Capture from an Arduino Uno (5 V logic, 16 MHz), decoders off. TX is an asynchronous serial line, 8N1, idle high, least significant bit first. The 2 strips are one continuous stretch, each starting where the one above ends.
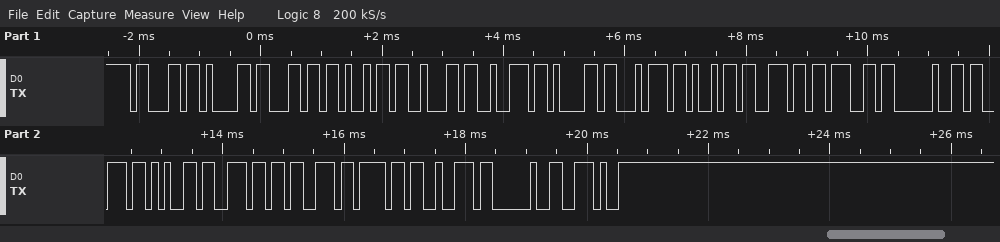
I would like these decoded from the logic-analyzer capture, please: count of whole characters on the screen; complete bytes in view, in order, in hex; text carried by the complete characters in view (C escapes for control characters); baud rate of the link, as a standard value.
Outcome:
20
0x63 0x61 0x6C 0x69 0x62 0x72 0x61 0x74 0x69 0x6E 0x67 0x20 0x73 0x65 0x6E 0x73 0x6F 0x72 0x20 0x2E
"calibrating sensor ."
9600 baud
